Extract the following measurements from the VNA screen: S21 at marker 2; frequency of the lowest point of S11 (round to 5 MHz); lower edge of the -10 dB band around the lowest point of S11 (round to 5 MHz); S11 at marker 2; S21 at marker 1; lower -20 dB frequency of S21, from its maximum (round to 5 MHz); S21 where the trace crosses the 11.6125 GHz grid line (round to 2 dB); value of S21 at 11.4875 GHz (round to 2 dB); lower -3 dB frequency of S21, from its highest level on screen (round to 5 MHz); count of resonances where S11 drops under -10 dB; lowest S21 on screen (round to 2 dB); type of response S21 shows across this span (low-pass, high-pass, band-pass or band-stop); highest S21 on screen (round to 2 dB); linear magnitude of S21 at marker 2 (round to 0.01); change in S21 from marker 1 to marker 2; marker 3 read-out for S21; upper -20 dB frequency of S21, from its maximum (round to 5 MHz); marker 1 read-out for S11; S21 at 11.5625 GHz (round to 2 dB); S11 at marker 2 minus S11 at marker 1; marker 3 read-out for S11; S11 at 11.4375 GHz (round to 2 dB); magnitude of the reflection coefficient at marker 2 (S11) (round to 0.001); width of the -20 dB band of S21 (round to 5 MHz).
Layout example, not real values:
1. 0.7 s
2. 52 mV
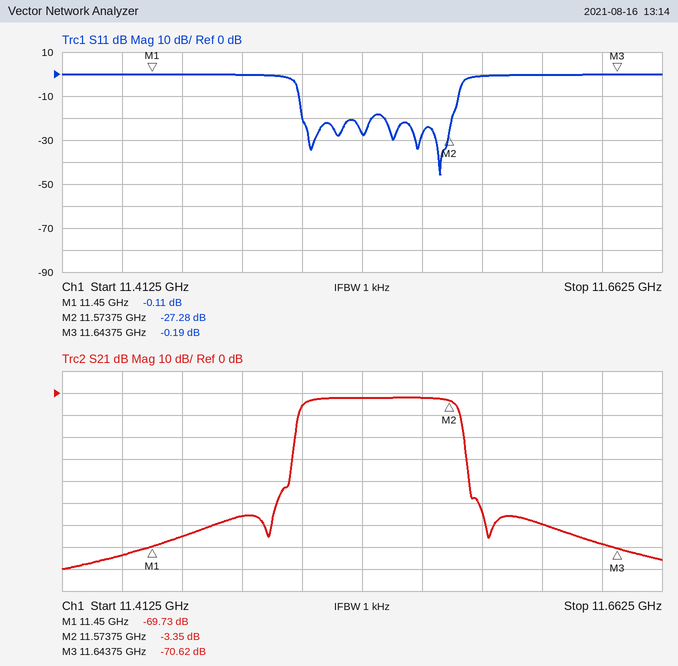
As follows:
1. -3.35 dB
2. 11.570 GHz
3. 11.510 GHz
4. -27.28 dB
5. -69.73 dB
6. 11.510 GHz
7. -60 dB
8. -56 dB
9. 11.515 GHz
10. 6
11. -80 dB
12. band-pass
13. -2 dB
14. 0.68
15. 66.38 dB
16. -70.62 dB
17. 11.580 GHz
18. -0.11 dB
19. -2 dB
20. -27.17 dB
21. -0.19 dB
22. 0 dB
23. 0.043
24. 70 MHz
